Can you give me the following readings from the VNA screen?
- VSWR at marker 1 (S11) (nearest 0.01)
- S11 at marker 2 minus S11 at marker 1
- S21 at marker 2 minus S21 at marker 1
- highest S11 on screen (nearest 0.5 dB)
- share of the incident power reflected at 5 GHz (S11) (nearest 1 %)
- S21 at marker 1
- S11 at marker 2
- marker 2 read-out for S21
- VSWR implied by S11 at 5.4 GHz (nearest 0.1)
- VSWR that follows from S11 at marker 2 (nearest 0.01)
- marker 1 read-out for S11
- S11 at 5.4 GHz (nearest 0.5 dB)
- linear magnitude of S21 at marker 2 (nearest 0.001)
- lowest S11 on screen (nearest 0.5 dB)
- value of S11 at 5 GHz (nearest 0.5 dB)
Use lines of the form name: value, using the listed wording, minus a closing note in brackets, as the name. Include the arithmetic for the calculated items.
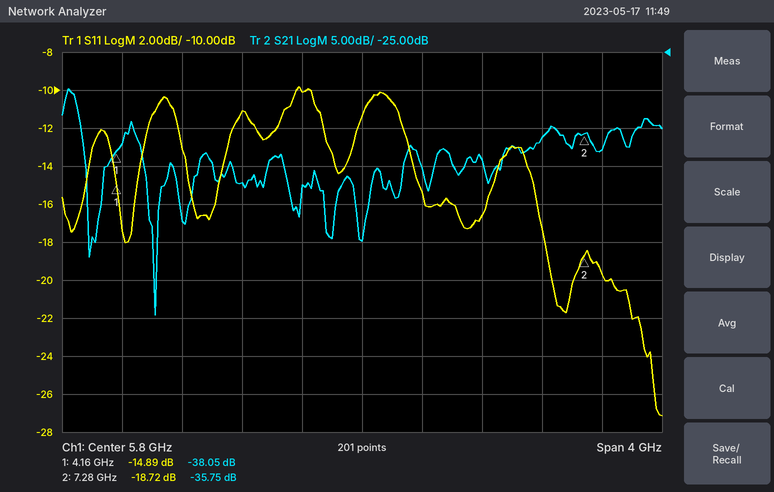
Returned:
VSWR at marker 1 (S11): (1 + 0.1801)/(1 − 0.1801) ≈ 1.44
S11 at marker 2 minus S11 at marker 1: -18.72 − (-14.89) = -3.83 dB
S21 at marker 2 minus S21 at marker 1: -35.75 − (-38.05) = 2.30 dB
highest S11 on screen: -10.0 dB
share of the incident power reflected at 5 GHz (S11): 10^(-11/10) ≈ 8 %
S21 at marker 1: -38.05 dB
S11 at marker 2: -18.72 dB
marker 2 read-out for S21: -35.75 dB
VSWR implied by S11 at 5.4 GHz: |Γ| = 10^(-10/20) = 0.3162; VSWR = (1 + 0.3162)/(1 − 0.3162) ≈ 1.9
VSWR that follows from S11 at marker 2: (1 + 0.1159)/(1 − 0.1159) ≈ 1.26
marker 1 read-out for S11: -14.89 dB
S11 at 5.4 GHz: -10.0 dB
linear magnitude of S21 at marker 2: 10^(-35.75/20) ≈ 0.016
lowest S11 on screen: -27.0 dB
value of S11 at 5 GHz: -11.0 dB
